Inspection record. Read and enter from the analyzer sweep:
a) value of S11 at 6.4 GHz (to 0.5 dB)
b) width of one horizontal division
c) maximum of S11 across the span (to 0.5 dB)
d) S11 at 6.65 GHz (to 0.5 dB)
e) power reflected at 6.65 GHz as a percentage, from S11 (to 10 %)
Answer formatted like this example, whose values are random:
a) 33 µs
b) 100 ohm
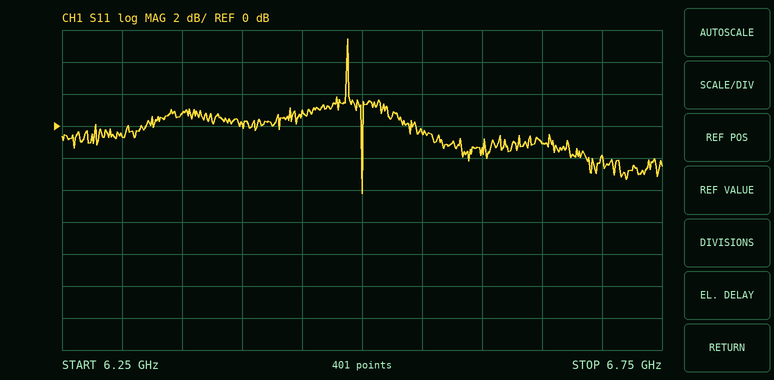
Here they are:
a) 0.0 dB
b) 50 MHz
c) 5.5 dB
d) -1.0 dB
e) 80 %
